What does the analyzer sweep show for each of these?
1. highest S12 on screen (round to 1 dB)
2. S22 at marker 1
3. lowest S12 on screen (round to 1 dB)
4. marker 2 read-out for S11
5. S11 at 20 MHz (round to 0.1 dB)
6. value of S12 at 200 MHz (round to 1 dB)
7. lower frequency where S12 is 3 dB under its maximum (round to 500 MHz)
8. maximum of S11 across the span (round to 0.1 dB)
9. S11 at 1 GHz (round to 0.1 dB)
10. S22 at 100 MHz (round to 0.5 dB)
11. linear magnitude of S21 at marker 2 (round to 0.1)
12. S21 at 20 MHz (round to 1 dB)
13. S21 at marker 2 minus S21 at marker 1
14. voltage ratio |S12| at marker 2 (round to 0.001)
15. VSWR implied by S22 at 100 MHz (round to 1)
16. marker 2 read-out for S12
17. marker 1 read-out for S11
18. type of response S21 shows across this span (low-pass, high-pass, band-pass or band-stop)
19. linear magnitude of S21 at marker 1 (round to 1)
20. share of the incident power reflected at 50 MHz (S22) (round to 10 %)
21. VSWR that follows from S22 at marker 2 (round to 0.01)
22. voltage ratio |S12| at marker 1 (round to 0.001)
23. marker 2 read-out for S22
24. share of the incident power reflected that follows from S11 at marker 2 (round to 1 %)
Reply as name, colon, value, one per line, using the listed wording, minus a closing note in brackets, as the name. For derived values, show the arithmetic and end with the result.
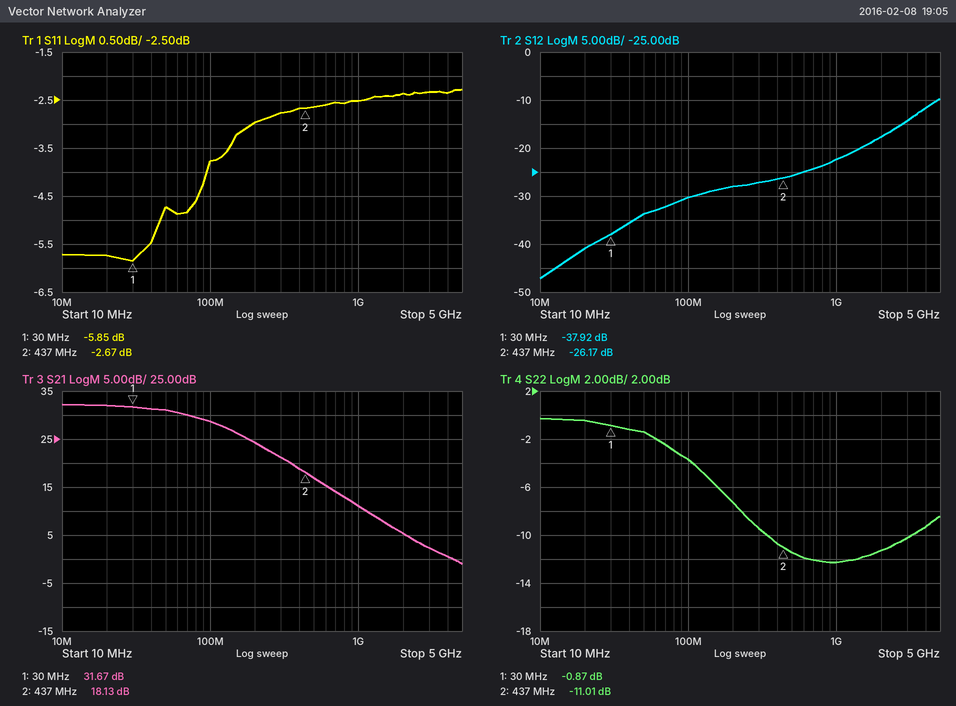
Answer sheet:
highest S12 on screen: -10 dB
S22 at marker 1: -0.87 dB
lowest S12 on screen: -47 dB
marker 2 read-out for S11: -2.67 dB
S11 at 20 MHz: -5.7 dB
value of S12 at 200 MHz: -28 dB
lower frequency where S12 is 3 dB under its maximum: 3.5 GHz
maximum of S11 across the span: -2.3 dB
S11 at 1 GHz: -2.5 dB
S22 at 100 MHz: -3.5 dB
linear magnitude of S21 at marker 2: 10^(18.13/20) ≈ 8.1
S21 at 20 MHz: 32 dB
S21 at marker 2 minus S21 at marker 1: 18.13 − (31.67) = -13.54 dB
voltage ratio |S12| at marker 2: 10^(-26.17/20) ≈ 0.049
VSWR implied by S22 at 100 MHz: |Γ| = 10^(-3.5/20) = 0.6683; VSWR = (1 + 0.6683)/(1 − 0.6683) ≈ 5
marker 2 read-out for S12: -26.17 dB
marker 1 read-out for S11: -5.85 dB
type of response S21 shows across this span: low-pass
linear magnitude of S21 at marker 1: 10^(31.67/20) ≈ 38
share of the incident power reflected at 50 MHz (S22): 10^(-1.5/10) ≈ 70.8 %, so 70 % to the nearest 10 %
VSWR that follows from S22 at marker 2: (1 + 0.2815)/(1 − 0.2815) ≈ 1.78
voltage ratio |S12| at marker 1: 10^(-37.92/20) ≈ 0.013
marker 2 read-out for S22: -11.01 dB
share of the incident power reflected that follows from S11 at marker 2: 10^(-2.67/10) ≈ 54 %
